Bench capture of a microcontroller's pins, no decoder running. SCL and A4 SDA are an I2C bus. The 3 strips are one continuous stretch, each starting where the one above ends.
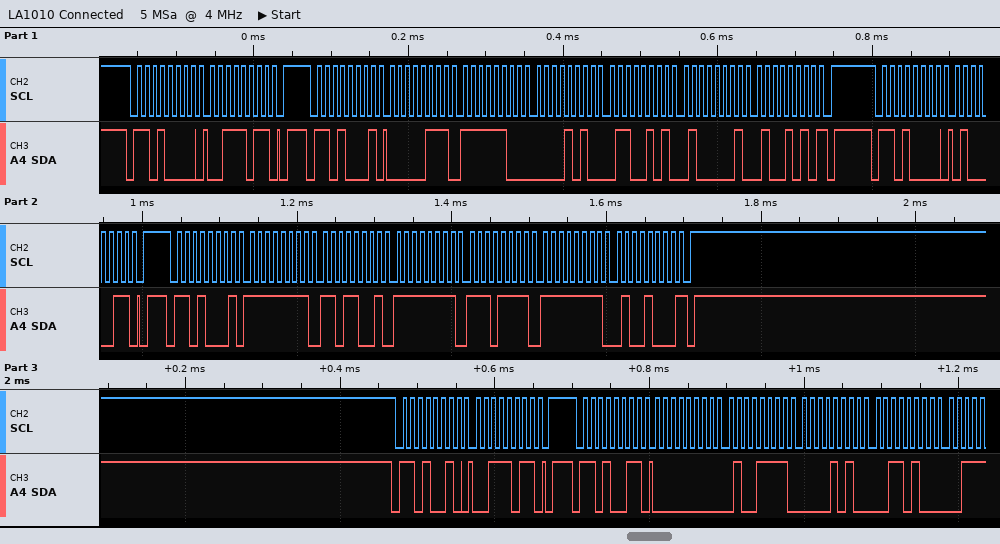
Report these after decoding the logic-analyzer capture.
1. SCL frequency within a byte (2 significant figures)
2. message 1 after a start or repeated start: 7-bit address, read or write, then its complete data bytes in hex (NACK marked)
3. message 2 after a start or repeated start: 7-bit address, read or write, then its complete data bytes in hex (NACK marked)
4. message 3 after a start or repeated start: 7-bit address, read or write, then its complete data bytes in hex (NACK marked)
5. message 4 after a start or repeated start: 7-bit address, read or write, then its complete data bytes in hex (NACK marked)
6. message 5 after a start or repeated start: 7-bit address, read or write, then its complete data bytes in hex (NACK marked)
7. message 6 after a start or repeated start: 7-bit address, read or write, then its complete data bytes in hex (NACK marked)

100 kHz
0x68 write: 3B
0x68 read: 07 FC 0A 65 41 4A NACK
0x68 write: 43
0x68 read: FF D9 FF EF FF 48 NACK
0x69 write: 3B
0x69 read: 00 4F 0A 34
